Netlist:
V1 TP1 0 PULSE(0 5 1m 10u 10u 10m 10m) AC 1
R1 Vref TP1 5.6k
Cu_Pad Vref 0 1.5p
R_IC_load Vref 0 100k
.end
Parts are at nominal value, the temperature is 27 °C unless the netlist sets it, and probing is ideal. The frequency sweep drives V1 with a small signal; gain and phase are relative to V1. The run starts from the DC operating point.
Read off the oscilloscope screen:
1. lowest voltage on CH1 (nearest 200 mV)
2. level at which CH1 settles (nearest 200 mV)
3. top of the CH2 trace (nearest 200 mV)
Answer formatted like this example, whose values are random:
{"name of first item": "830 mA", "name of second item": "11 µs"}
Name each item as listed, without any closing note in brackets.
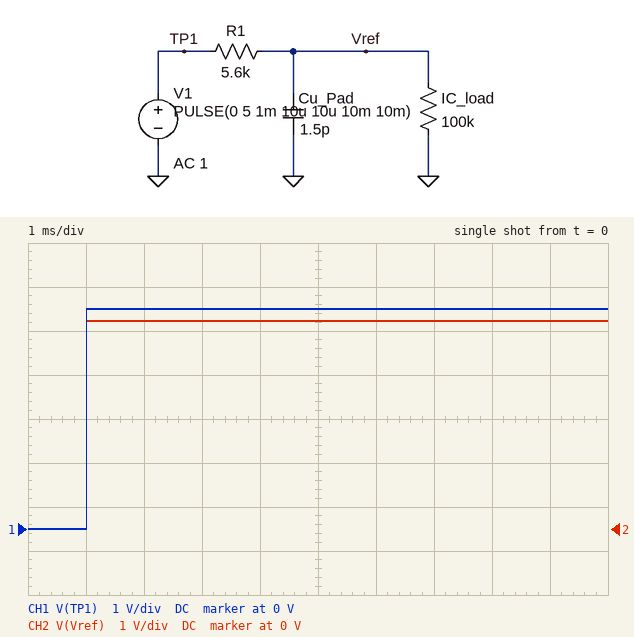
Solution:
{"lowest voltage on CH1": "0 V", "level at which CH1 settles": "5.0 V", "top of the CH2 trace": "4.8 V"}
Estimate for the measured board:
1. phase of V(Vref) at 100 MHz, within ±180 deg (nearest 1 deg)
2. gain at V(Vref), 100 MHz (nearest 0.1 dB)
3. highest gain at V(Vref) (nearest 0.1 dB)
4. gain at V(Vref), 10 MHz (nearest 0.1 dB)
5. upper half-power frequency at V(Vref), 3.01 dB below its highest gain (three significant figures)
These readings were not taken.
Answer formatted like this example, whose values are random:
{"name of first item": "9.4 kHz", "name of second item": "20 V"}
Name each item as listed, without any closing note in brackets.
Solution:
{"phase of V(Vref) at 100 MHz, within ±180 deg": "-79 deg", "gain at V(Vref), 100 MHz": "-14.6 dB", "highest gain at V(Vref)": "-0.5 dB", "gain at V(Vref), 10 MHz": "-1.4 dB", "upper half-power frequency at V(Vref), 3.01 dB below its highest gain": "20.0 MHz"}
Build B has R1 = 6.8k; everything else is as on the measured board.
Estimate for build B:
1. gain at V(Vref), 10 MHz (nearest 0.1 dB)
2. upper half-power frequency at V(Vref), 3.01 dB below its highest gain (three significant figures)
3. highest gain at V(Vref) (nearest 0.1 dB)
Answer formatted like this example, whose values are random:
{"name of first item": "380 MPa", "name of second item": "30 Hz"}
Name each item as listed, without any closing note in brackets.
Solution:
{"gain at V(Vref), 10 MHz": "-1.9 dB", "upper half-power frequency at V(Vref), 3.01 dB below its highest gain": "16.7 MHz", "highest gain at V(Vref)": "-0.6 dB"}
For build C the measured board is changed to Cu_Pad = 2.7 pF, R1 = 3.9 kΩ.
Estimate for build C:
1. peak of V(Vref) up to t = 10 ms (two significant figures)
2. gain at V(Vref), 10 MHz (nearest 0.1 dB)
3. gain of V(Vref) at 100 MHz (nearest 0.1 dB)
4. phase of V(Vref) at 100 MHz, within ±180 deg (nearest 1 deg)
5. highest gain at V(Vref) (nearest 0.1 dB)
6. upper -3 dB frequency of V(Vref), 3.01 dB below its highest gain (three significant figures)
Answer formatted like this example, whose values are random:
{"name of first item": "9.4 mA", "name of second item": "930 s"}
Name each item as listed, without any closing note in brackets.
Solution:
{"peak of V(Vref) up to t = 10 ms": "4.8 V", "gain at V(Vref), 10 MHz": "-1.8 dB", "gain of V(Vref) at 100 MHz": "-16.5 dB", "phase of V(Vref) at 100 MHz, within ±180 deg": "-81 deg", "highest gain at V(Vref)": "-0.3 dB", "upper -3 dB frequency of V(Vref), 3.01 dB below its highest gain": "15.7 MHz"}
